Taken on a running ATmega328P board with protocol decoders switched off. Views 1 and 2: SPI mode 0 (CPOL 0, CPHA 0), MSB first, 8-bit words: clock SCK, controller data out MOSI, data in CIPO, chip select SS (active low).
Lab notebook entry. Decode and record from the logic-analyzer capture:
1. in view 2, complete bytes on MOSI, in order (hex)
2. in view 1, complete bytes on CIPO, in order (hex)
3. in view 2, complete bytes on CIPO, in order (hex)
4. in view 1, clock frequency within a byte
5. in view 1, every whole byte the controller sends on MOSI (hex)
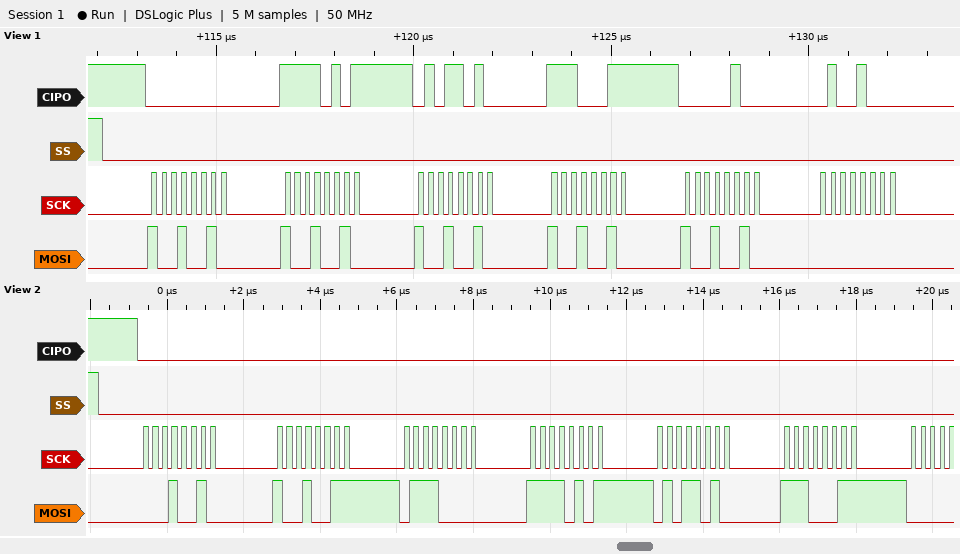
0x12 0x93 0x70 0xF5 0x5A 0xE3
00 F5 5A E3 04 48
0x00 0x00 0x00 0x00 0x00 0x00
4 MHz
92 92 92 92 92 00
